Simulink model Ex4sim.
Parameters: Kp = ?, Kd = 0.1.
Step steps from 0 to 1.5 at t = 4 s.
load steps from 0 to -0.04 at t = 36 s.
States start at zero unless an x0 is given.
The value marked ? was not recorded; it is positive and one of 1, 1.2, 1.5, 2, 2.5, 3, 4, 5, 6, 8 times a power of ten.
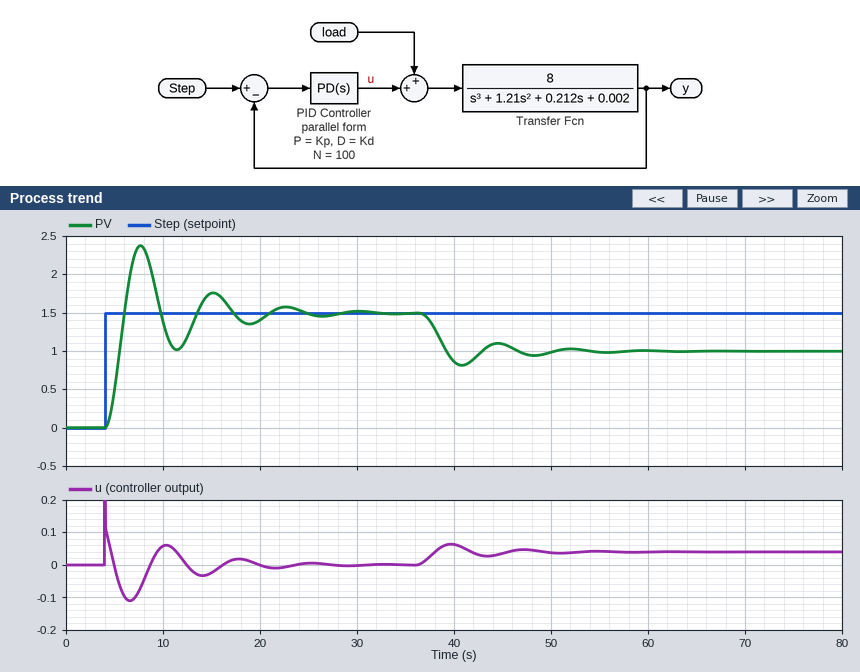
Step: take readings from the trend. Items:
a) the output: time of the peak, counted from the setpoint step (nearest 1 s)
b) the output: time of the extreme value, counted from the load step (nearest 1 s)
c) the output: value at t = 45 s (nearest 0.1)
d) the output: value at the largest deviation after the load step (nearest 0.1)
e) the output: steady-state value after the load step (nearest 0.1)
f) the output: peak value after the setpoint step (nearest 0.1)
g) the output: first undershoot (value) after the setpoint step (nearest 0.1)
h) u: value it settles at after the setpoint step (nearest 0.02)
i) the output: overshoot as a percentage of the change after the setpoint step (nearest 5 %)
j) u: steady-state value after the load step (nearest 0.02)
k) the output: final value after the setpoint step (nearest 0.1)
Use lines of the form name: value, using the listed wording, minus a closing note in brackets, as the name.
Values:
the output: time of the peak, counted from the setpoint step: 4 s
the output: time of the extreme value, counted from the load step: 5 s
the output: value at t = 45 s: 1.1
the output: value at the largest deviation after the load step: 0.8
the output: steady-state value after the load step: 1.0
the output: peak value after the setpoint step: 2.4
the output: first undershoot (value) after the setpoint step: 1.0
u: value it settles at after the setpoint step: 0.00
the output: overshoot as a percentage of the change after the setpoint step: 60 %
u: steady-state value after the load step: 0.04
the output: final value after the setpoint step: 1.5
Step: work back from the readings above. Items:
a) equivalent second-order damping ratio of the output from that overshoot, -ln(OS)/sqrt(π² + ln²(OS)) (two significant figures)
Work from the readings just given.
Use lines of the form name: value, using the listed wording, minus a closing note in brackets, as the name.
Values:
equivalent second-order damping ratio of the output from that overshoot, -ln(OS)/sqrt(π² + ln²(OS)): 0.16
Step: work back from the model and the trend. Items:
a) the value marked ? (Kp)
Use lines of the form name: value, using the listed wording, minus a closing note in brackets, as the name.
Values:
the value marked ?: 0.08
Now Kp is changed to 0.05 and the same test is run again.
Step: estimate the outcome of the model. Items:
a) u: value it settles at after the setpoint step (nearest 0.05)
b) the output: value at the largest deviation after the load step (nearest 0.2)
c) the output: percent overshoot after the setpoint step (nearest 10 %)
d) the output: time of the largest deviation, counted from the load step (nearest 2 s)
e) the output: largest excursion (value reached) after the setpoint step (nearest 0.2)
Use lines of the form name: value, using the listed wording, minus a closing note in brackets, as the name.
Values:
u: value it settles at after the setpoint step: 0.00
the output: value at the largest deviation after the load step: 0.6
the output: percent overshoot after the setpoint step: 40 %
the output: time of the largest deviation, counted from the load step: 6 s
the output: largest excursion (value reached) after the setpoint step: 2.0
